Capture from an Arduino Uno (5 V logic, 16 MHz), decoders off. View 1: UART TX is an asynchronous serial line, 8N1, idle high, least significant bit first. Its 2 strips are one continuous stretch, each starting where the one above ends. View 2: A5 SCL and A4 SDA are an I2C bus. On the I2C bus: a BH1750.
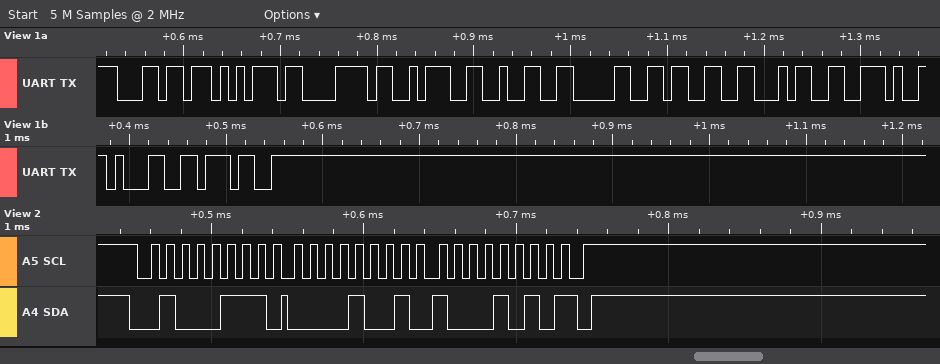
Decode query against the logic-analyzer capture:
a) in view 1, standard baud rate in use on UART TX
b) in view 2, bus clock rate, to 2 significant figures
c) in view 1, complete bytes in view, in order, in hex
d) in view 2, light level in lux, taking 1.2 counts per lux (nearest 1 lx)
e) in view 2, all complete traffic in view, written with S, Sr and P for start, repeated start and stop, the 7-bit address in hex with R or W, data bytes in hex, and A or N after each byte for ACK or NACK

115200 baud
100 kHz
6C 75 78 3A 32 30 33 34 2E 31 37
2035 lx
S 23R A 09 A 8A N P
